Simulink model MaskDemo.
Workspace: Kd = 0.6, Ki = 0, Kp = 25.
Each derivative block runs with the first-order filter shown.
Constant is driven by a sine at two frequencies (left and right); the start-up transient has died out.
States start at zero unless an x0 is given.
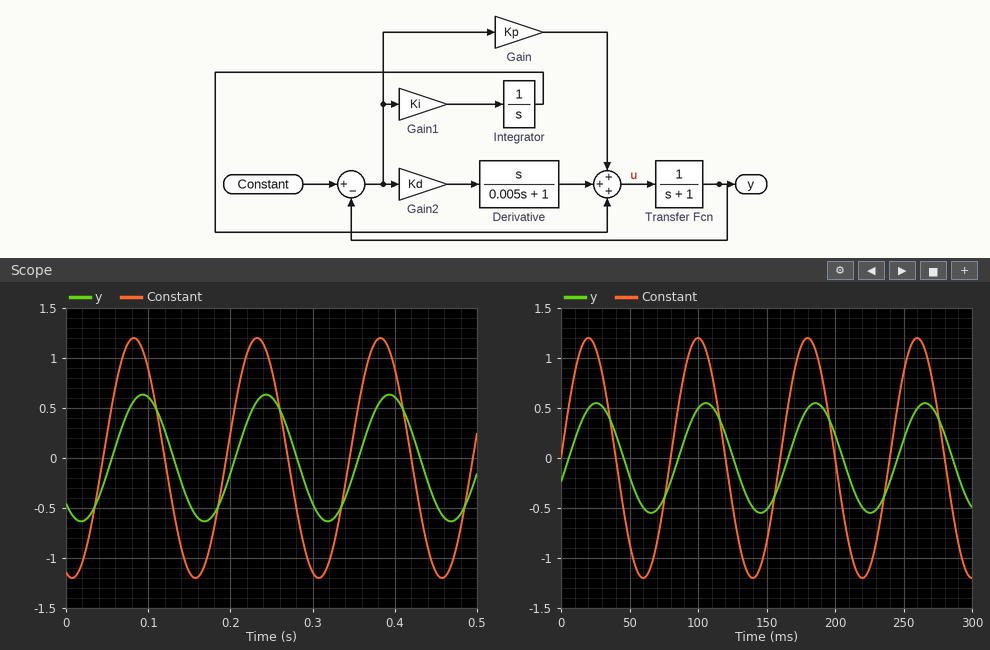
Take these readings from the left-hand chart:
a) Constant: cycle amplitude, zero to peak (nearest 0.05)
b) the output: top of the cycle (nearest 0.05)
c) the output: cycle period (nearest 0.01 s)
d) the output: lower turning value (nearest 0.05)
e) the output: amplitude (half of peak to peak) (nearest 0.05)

1.20
0.65
0.15 s
-0.65
0.65
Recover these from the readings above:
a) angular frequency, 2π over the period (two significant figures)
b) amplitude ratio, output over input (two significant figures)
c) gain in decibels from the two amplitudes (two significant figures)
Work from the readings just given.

42 rad/s
0.54
-5.3 dB
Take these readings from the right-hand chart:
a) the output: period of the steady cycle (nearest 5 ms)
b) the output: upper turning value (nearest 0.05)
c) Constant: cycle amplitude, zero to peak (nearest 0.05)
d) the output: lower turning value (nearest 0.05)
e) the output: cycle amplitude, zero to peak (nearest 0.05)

80 ms
0.55
1.20
-0.55
0.55
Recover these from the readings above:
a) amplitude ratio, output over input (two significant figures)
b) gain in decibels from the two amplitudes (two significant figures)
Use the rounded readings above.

0.46
-6.8 dB
